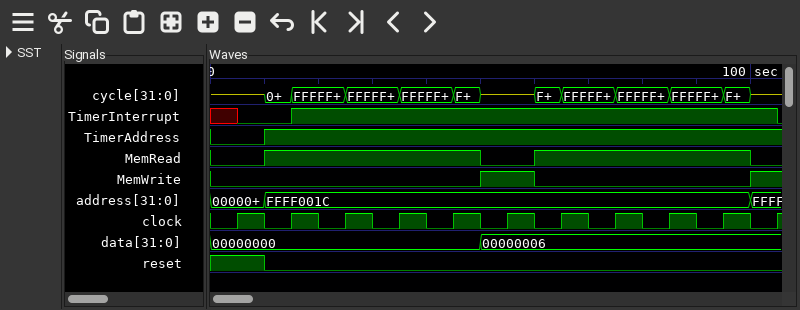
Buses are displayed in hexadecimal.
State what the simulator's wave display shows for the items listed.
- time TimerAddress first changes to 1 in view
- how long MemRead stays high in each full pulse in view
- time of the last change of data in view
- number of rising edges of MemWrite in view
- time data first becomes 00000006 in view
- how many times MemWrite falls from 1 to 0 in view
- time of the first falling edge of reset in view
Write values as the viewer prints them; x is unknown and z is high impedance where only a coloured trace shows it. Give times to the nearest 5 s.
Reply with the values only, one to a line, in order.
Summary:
10 s
40 s, 40 s
50 s
2
50 s
1
10 s
